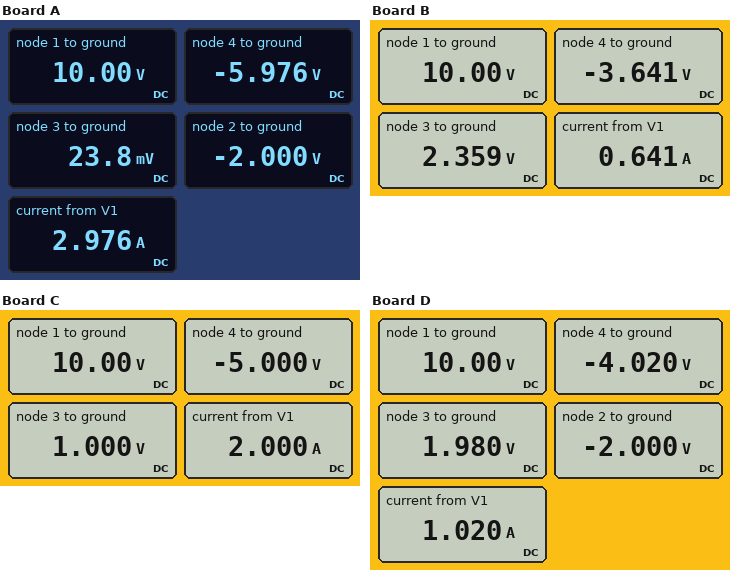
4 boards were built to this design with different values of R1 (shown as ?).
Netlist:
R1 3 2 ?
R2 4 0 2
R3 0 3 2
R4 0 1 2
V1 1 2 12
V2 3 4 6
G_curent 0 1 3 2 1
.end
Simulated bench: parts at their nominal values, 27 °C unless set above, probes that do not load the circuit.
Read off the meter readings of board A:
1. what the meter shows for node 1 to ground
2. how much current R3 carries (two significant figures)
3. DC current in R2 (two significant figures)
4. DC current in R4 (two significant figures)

10.00 V
12 mA
3.0 A
5.0 A
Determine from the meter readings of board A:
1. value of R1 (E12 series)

0.68 Ω
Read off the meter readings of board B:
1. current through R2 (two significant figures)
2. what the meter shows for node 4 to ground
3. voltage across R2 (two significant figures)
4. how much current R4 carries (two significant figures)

1.8 A
-3.641 V
3.6 V
5.0 A
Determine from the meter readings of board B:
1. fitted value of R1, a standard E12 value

6.8 Ω
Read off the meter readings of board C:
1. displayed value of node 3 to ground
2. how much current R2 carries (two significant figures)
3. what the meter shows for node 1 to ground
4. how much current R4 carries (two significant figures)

1.000 V
2.5 A
10.00 V
5.0 A
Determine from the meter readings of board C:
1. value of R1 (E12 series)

1.5 Ω
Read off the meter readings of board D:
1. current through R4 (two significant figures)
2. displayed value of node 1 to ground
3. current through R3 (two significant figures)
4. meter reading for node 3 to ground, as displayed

5.0 A
10.00 V
990 mA
1.980 V
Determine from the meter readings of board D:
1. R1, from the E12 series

3.9 Ω
